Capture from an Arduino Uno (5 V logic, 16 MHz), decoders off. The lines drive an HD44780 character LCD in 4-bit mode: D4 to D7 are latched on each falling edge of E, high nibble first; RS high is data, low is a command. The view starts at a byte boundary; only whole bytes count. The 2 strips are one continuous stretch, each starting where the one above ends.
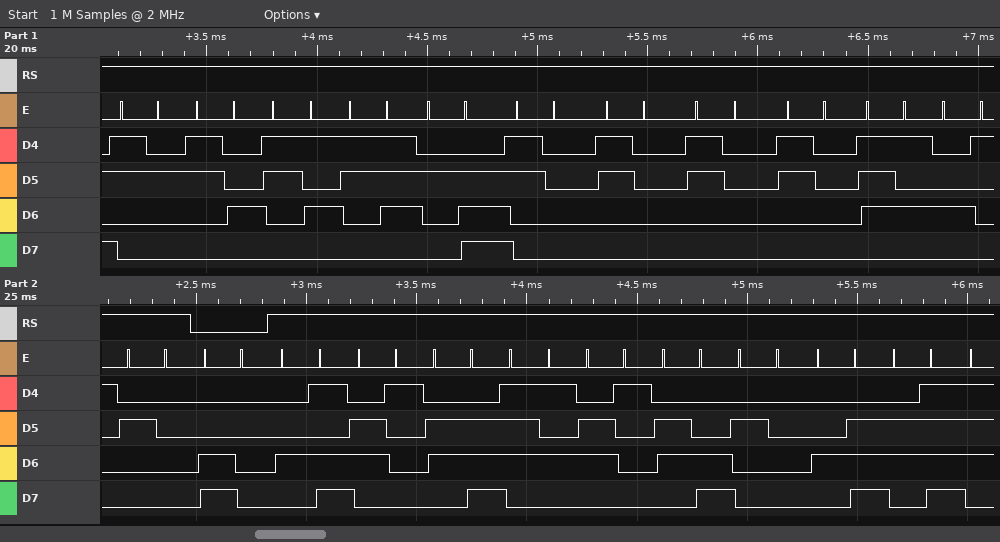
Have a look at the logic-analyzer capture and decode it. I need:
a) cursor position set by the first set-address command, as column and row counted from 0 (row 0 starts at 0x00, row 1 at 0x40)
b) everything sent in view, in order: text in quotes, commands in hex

column 0, row 1
"2457.0000uA " 0xC0 "Manual No"
